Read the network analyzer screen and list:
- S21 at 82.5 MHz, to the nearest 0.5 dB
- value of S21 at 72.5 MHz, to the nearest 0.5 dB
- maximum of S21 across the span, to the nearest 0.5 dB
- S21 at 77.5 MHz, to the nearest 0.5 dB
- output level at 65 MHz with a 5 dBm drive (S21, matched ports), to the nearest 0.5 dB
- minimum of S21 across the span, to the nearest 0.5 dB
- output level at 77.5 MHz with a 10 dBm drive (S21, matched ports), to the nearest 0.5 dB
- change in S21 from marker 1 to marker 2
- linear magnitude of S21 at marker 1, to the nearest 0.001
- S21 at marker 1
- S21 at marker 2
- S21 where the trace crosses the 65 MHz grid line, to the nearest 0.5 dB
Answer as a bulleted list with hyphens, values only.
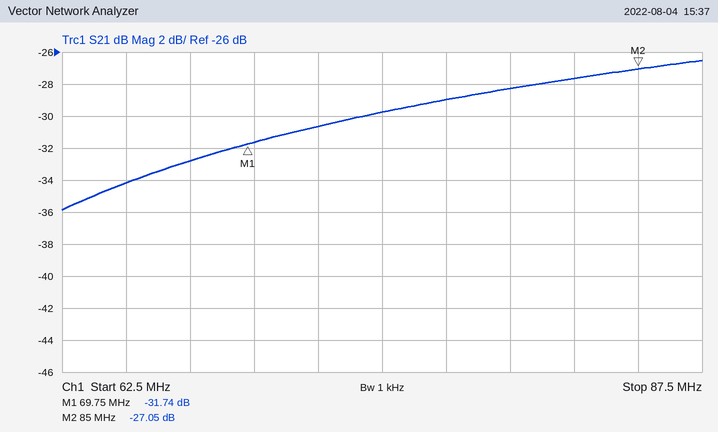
- -27.5 dB
- -30.5 dB
- -26.5 dB
- -29.0 dB
- -29.0 dBm
- -36.0 dB
- -19.0 dBm
- 4.69 dB
- 0.026
- -31.74 dB
- -27.05 dB
- -34.0 dB
